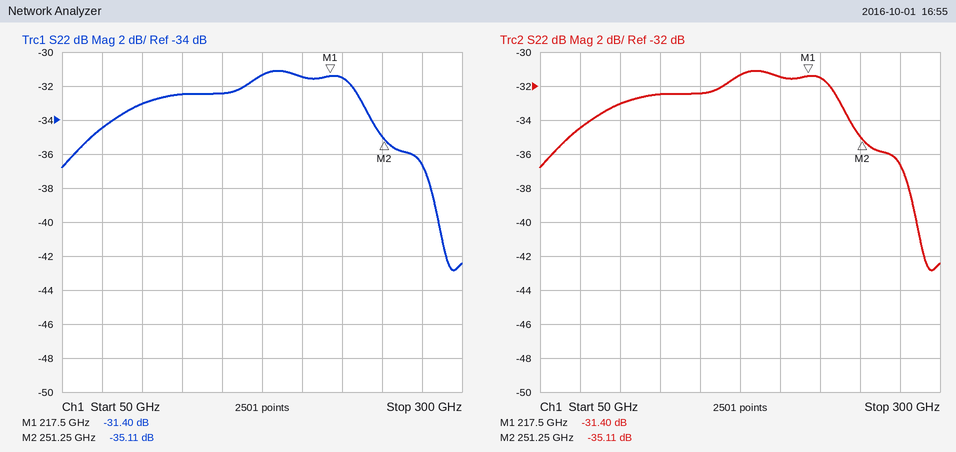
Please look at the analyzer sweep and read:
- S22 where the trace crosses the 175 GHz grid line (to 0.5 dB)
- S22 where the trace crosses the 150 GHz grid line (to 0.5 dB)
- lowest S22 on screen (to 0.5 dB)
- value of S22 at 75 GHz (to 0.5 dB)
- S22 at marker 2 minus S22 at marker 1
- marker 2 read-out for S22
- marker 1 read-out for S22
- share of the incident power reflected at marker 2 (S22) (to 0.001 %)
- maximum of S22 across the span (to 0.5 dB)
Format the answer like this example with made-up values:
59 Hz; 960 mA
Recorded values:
-31.5 dB; -32.5 dB; -43.0 dB; -34.5 dB; -3.71 dB; -35.11 dB; -31.40 dB; 0.031 %; -31.0 dB
